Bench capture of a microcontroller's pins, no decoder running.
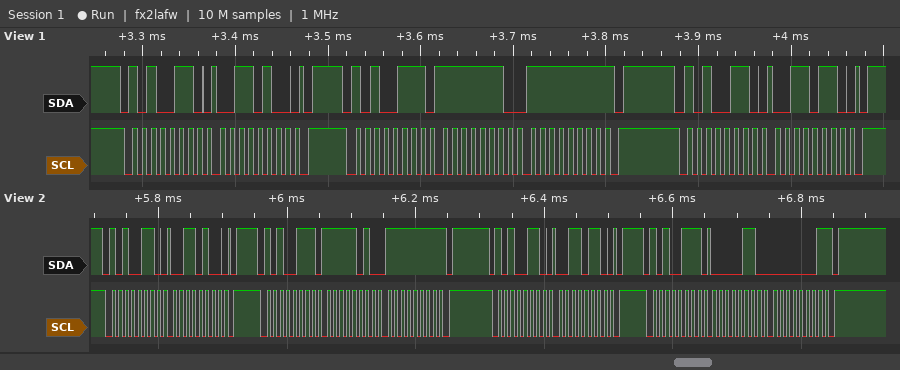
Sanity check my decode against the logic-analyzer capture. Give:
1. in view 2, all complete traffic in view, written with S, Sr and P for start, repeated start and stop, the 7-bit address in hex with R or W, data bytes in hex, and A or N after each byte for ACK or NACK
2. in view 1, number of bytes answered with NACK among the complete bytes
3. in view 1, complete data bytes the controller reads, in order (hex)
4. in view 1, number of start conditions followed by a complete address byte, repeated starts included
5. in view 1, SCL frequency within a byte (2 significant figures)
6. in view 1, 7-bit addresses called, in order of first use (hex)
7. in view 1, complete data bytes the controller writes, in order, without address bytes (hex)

S 53W A 34 A P S 53R A FA A FF N P S 53W A 36 A P S 53R A 06 A 01 N P
1
FE FF
3
100 kHz
0x53
34 36
